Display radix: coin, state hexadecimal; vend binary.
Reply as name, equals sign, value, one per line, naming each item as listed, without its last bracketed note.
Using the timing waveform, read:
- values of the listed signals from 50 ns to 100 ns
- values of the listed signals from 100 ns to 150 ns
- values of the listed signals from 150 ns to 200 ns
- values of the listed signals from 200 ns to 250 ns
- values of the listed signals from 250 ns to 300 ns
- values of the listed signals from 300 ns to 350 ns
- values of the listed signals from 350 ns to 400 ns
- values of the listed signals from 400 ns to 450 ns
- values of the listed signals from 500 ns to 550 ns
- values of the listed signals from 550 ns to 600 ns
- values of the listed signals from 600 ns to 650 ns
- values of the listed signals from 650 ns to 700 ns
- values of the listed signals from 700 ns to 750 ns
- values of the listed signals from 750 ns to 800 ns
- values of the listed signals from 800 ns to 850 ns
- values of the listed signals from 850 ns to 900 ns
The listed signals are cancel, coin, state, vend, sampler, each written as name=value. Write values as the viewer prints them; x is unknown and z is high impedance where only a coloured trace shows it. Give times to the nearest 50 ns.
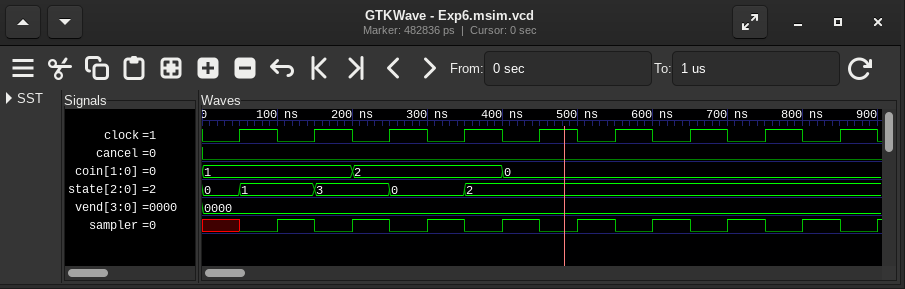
values of the listed signals from 50 ns to 100 ns = cancel=0, coin=1, state=1, vend=0000, sampler=0
values of the listed signals from 100 ns to 150 ns = cancel=0, coin=1, state=1, vend=0000, sampler=1
values of the listed signals from 150 ns to 200 ns = cancel=0, coin=1, state=3, vend=0000, sampler=0
values of the listed signals from 200 ns to 250 ns = cancel=0, coin=2, state=3, vend=0000, sampler=1
values of the listed signals from 250 ns to 300 ns = cancel=0, coin=2, state=0, vend=0000, sampler=0
values of the listed signals from 300 ns to 350 ns = cancel=0, coin=2, state=0, vend=0000, sampler=1
values of the listed signals from 350 ns to 400 ns = cancel=0, coin=2, state=2, vend=0000, sampler=0
values of the listed signals from 400 ns to 450 ns = cancel=0, coin=0, state=2, vend=0000, sampler=1
values of the listed signals from 500 ns to 550 ns = cancel=0, coin=0, state=2, vend=0000, sampler=1
values of the listed signals from 550 ns to 600 ns = cancel=0, coin=0, state=2, vend=0000, sampler=0
values of the listed signals from 600 ns to 650 ns = cancel=0, coin=0, state=2, vend=0000, sampler=1
values of the listed signals from 650 ns to 700 ns = cancel=0, coin=0, state=2, vend=0000, sampler=0
values of the listed signals from 700 ns to 750 ns = cancel=0, coin=0, state=2, vend=0000, sampler=1
values of the listed signals from 750 ns to 800 ns = cancel=0, coin=0, state=2, vend=0000, sampler=0
values of the listed signals from 800 ns to 850 ns = cancel=0, coin=0, state=2, vend=0000, sampler=1
values of the listed signals from 850 ns to 900 ns = cancel=0, coin=0, state=2, vend=0000, sampler=0
